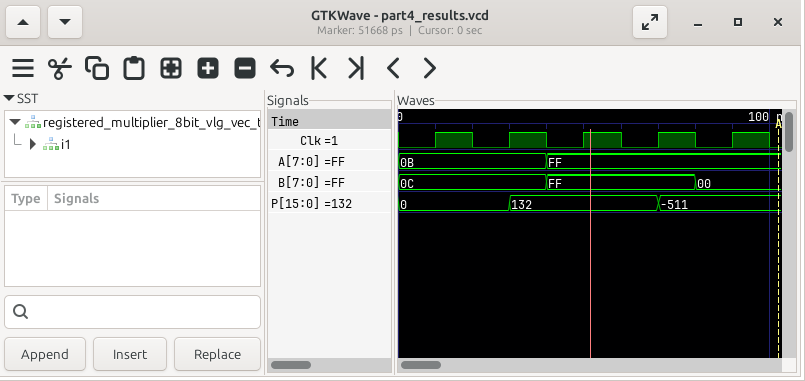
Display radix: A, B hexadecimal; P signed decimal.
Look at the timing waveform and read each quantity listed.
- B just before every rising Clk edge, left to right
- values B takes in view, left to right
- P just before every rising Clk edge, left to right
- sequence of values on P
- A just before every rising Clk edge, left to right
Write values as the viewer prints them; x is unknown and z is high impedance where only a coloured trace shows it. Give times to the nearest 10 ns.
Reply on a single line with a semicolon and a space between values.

0C, 0C, FF, FF, 00; 0C, FF, 00; 0, 0, 132, 132, -511; 0, 132, -511; 0B, 0B, FF, FF, FF
